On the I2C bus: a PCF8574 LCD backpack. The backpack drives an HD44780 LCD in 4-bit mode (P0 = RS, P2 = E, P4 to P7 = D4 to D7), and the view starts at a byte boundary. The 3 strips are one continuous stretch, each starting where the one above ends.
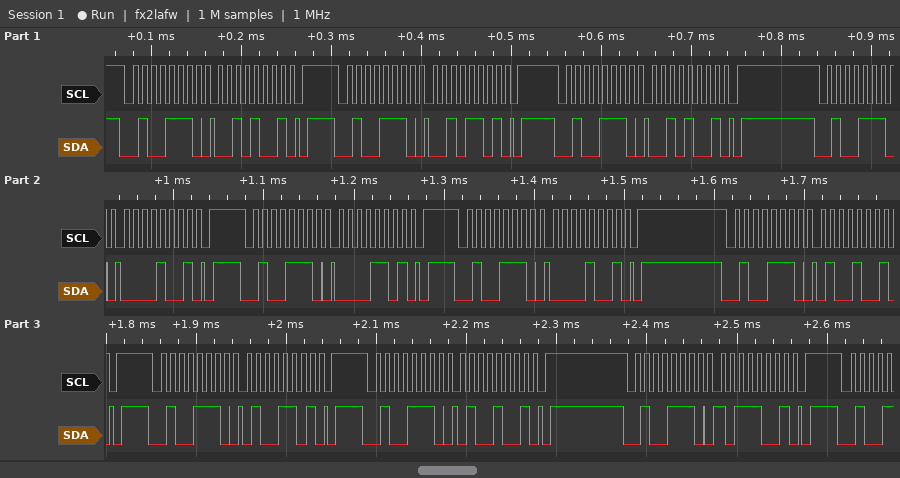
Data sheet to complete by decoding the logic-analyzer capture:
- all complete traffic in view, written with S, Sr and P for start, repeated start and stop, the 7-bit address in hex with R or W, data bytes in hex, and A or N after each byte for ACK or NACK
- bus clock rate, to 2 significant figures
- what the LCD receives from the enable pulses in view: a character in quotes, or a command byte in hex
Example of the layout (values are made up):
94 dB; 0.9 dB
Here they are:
S 27W A 29 A P S 27W A 2D A P S 27W A 29 A P S 27W A 09 A P S 27W A 0D A P S 27W A 09 A P S 27W A 49 A P S 27W A 4D A P S 27W A 49 A P S 27W A B9 A P; 100 kHz; ' '
